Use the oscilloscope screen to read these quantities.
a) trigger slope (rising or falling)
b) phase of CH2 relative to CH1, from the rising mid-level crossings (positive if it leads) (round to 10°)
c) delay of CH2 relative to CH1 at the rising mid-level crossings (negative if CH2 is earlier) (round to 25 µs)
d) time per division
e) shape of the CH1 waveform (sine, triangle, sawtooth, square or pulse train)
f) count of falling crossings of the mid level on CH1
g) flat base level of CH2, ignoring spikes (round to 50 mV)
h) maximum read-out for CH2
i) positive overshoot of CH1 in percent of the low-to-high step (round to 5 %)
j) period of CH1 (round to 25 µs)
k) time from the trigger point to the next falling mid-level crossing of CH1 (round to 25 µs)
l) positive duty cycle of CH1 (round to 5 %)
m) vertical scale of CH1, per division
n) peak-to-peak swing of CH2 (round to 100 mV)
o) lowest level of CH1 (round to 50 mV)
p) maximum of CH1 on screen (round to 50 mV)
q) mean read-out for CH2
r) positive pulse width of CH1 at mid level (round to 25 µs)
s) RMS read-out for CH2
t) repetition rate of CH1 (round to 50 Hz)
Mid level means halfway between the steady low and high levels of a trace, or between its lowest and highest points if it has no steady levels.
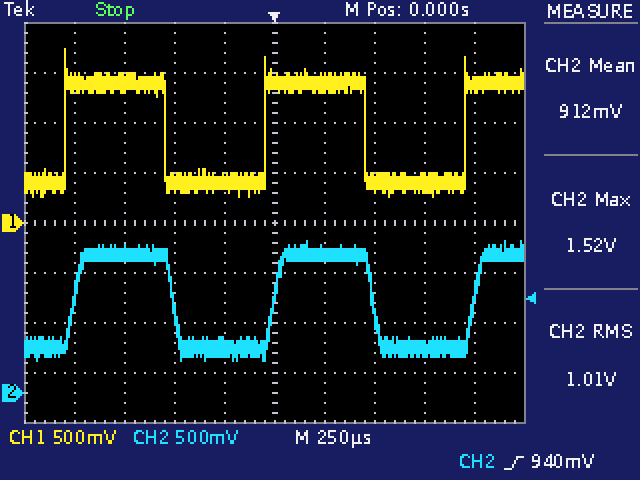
rising
-20°
+50 µs
250 µs
square
2
450 mV
1.52 V
35 %
1.000 ms
450 µs
50 %
500 mV
1.20 V
250 mV
1.75 V
912 mV
500 µs
1.01 V
1.00 kHz
